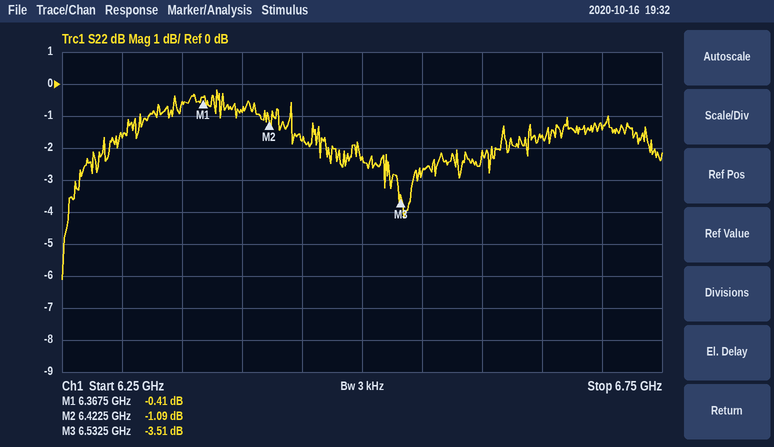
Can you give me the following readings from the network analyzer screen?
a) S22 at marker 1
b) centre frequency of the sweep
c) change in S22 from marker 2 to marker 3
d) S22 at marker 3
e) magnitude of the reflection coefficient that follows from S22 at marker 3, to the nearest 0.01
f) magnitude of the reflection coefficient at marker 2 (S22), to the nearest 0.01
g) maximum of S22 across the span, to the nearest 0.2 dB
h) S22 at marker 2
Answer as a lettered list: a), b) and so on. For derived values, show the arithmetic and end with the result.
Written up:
a) -0.41 dB
b) 6.5 GHz
c) -3.51 − (-1.09) = -2.42 dB
d) -3.51 dB
e) 10^(-3.51/20) ≈ 0.67
f) 10^(-1.09/20) ≈ 0.88
g) -0.2 dB
h) -1.09 dB
